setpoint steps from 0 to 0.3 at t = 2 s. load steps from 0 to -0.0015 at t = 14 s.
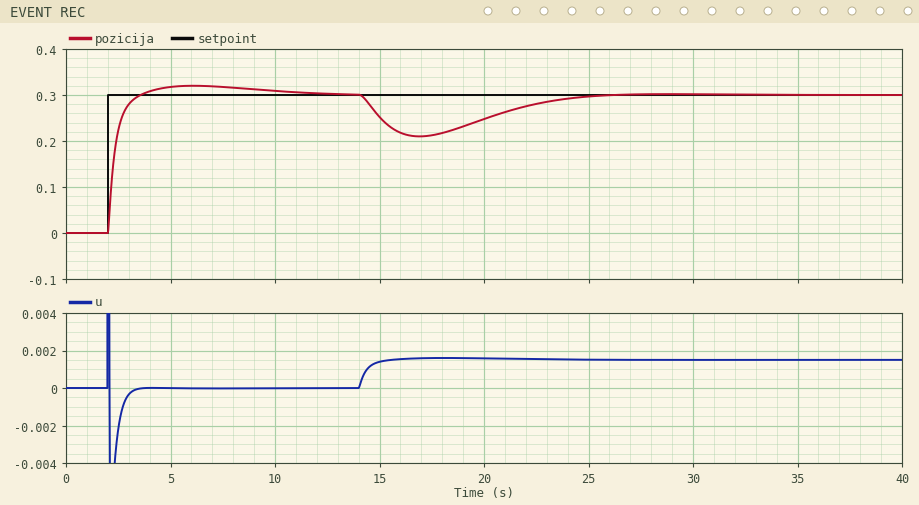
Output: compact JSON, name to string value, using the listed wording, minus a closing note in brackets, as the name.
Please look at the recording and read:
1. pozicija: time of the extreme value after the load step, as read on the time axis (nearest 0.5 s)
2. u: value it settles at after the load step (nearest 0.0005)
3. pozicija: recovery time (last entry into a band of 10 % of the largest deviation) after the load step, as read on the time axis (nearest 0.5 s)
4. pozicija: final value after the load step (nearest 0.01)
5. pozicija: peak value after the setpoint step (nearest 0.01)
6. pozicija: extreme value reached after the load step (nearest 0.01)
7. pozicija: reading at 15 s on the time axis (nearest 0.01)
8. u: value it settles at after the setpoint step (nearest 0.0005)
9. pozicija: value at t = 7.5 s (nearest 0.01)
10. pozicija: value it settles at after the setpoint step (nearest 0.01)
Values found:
{"pozicija: time of the extreme value after the load step, as read on the time axis": "17.0 s", "u: value it settles at after the load step": "0.0015", "pozicija: recovery time (last entry into a band of 10 % of the largest deviation) after the load step, as read on the time axis": "24.0 s", "pozicija: final value after the load step": "0.30", "pozicija: peak value after the setpoint step": "0.32", "pozicija: extreme value reached after the load step": "0.21", "pozicija: reading at 15 s on the time axis": "0.25", "u: value it settles at after the setpoint step": "0.0000", "pozicija: value at t = 7.5 s": "0.32", "pozicija: value it settles at after the setpoint step": "0.30"}
